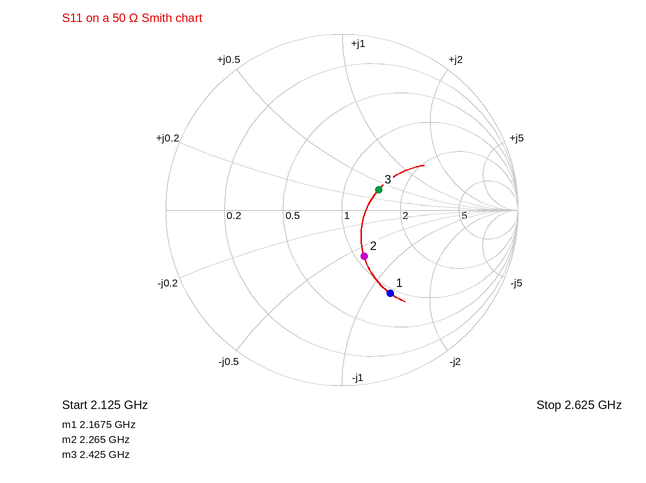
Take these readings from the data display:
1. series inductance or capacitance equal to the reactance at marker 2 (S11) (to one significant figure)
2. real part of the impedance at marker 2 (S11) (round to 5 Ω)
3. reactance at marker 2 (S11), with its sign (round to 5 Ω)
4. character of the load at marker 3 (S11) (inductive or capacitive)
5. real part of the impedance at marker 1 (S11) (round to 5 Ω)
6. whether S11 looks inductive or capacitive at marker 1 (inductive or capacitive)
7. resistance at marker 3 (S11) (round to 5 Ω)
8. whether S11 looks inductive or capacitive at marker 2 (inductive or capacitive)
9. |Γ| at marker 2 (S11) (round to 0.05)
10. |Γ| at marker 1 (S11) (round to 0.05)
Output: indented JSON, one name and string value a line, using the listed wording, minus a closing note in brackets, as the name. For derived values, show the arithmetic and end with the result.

{
  "series inductance or capacitance equal to the reactance at marker 2 (S11)": "C = 1/(2π × 2.265 GHz × 30 Ω) ≈ 2 pF",
  "real part of the impedance at marker 2 (S11)": "55 Ω",
  "reactance at marker 2 (S11), with its sign": "-30 Ω",
  "character of the load at marker 3 (S11)": "inductive",
  "real part of the impedance at marker 1 (S11)": "45 Ω",
  "whether S11 looks inductive or capacitive at marker 1": "capacitive",
  "resistance at marker 3 (S11)": "75 Ω",
  "whether S11 looks inductive or capacitive at marker 2": "capacitive",
  "|Γ| at marker 2 (S11)": "0.30",
  "|Γ| at marker 1 (S11)": "0.55"
}
